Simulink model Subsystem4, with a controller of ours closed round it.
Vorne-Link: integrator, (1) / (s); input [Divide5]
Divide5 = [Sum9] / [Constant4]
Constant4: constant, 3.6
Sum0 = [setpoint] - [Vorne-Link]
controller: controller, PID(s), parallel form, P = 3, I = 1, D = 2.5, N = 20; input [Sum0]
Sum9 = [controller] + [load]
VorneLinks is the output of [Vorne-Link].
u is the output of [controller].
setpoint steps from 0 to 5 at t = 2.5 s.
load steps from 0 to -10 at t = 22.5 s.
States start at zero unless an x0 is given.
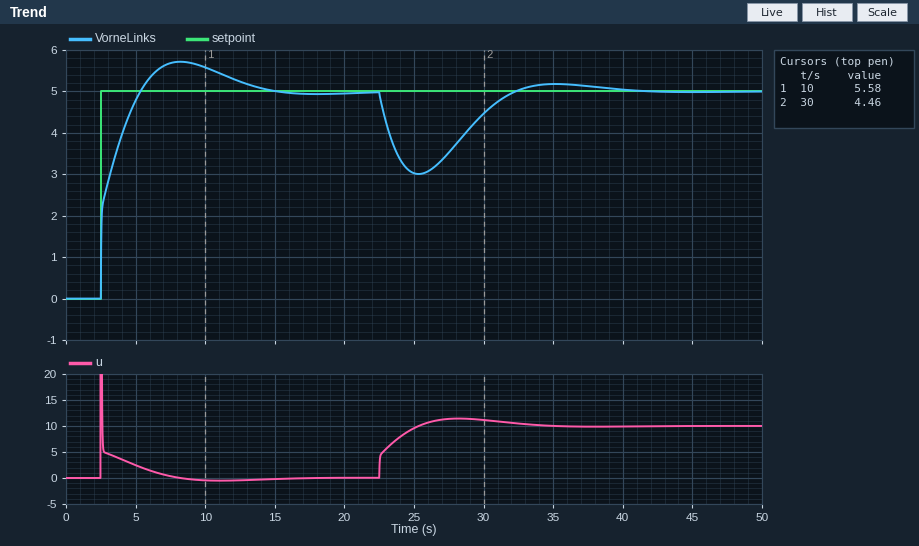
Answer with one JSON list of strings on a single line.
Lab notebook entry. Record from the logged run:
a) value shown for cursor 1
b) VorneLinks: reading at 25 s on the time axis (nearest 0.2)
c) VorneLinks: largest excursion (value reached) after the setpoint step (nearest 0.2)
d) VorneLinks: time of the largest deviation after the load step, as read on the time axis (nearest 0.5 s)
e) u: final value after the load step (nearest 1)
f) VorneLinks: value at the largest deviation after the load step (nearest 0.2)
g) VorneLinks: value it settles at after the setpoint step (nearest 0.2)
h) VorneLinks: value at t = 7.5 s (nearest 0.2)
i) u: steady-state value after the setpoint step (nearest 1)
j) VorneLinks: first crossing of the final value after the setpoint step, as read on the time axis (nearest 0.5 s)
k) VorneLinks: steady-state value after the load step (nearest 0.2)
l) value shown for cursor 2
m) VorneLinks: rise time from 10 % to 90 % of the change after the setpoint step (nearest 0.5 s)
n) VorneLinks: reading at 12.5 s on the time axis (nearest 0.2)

["5.58", "3.0", "5.8", "25.5 s", "10", "3.0", "5.0", "5.6", "0", "5.5 s", "5.0", "4.46", "2.0 s", "5.2"]
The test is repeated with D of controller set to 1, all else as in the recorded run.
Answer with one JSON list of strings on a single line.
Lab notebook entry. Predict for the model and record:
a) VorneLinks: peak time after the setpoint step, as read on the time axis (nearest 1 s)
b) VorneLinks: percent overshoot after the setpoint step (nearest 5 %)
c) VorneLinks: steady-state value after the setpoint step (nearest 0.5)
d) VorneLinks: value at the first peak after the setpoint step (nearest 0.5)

["7 s", "15 %", "5.0", "6.0"]
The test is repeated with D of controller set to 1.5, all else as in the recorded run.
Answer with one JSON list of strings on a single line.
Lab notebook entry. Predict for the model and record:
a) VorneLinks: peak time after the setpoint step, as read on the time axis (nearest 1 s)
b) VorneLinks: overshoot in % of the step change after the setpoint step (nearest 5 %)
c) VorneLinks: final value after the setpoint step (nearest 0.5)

["8 s", "15 %", "5.0"]
